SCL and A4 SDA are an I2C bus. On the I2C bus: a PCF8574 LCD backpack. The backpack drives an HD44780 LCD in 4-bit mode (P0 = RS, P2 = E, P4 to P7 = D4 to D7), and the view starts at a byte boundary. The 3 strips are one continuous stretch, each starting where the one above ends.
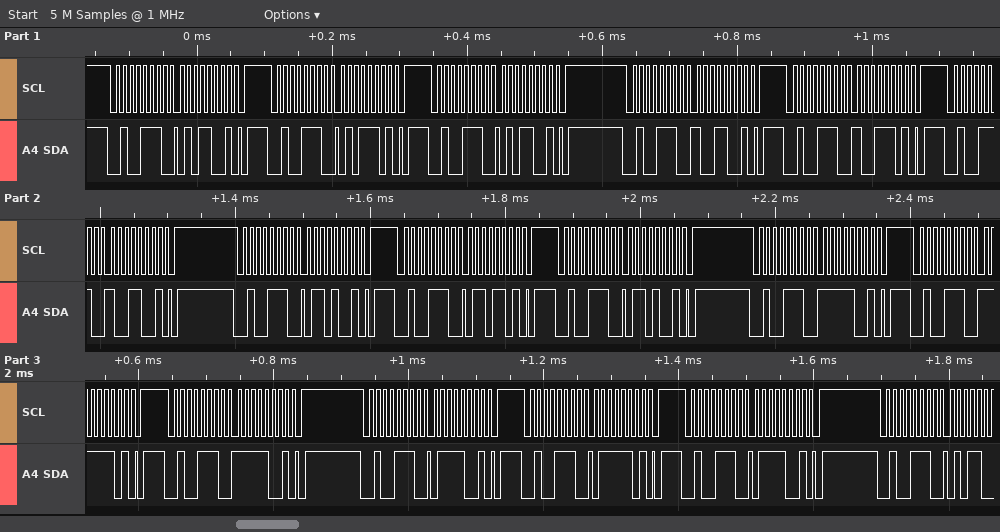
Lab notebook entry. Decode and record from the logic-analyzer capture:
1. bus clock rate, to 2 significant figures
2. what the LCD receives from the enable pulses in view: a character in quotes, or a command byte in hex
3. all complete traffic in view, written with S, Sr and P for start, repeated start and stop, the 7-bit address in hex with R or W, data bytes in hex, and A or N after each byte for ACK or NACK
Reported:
100 kHz
'Y' 'o'
S 27W A 59 A P S 27W A 5D A P S 27W A 59 A P S 27W A 99 A P S 27W A 9D A P S 27W A 99 A P S 27W A 69 A P S 27W A 6D A P S 27W A 69 A P S 27W A F9 A P S 27W A FD A P S 27W A F9 A P S 27W A 79 A P S 27W A 7D A P S 27W A 79 A P S 27W A
